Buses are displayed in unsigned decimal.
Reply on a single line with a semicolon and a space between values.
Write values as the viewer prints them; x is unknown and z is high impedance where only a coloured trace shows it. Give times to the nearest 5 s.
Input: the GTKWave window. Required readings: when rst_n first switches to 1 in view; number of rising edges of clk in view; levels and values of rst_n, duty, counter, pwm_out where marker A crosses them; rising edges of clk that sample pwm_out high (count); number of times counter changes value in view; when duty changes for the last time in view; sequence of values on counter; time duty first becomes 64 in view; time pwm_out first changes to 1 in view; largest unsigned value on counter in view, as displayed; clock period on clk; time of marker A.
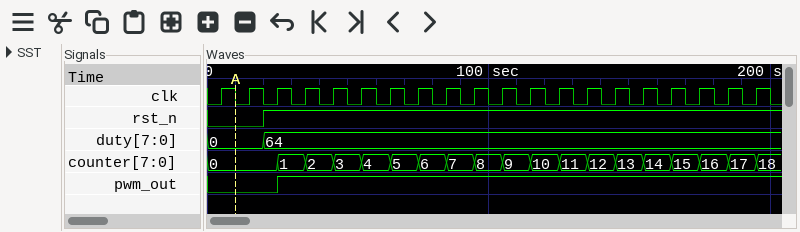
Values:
20 s; 20; rst_n=0, duty=0, counter=0, pwm_out=0; 17; 18; 20 s; 0, 1, 2, 3, 4, 5, 6, 7, 8, 9, 10, 11, 12, 13, 14, 15, 16, 17, 18; 20 s; 25 s; 18; 10 s; 10 s
